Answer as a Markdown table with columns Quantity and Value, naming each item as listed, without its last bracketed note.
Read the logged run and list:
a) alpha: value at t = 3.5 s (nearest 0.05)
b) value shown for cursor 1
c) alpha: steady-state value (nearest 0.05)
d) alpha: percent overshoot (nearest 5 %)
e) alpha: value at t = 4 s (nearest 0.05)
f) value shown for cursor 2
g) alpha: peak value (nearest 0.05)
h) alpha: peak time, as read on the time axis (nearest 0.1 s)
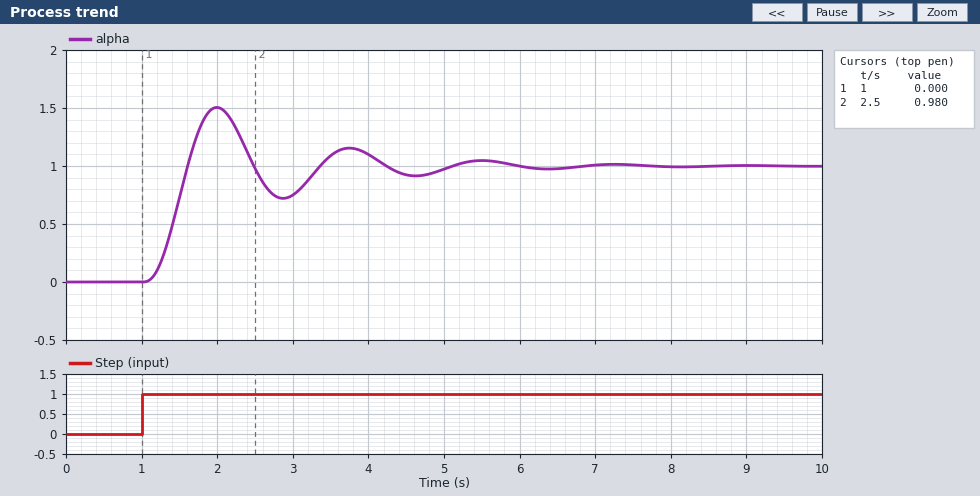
| Quantity | Value |
|---|---|
| alpha: value at t = 3.5 s | 1.10 |
| value shown for cursor 1 | 0.000 |
| alpha: steady-state value | 1.00 |
| alpha: percent overshoot | 50 % |
| alpha: value at t = 4 s | 1.10 |
| value shown for cursor 2 | 0.980 |
| alpha: peak value | 1.50 |
| alpha: peak time, as read on the time axis | 2.0 s |
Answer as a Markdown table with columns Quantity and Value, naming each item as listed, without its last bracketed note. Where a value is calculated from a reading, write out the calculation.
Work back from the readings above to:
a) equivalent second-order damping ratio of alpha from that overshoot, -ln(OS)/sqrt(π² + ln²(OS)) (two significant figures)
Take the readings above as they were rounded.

| Quantity | Value |
|---|---|
| equivalent second-order damping ratio of alpha from that overshoot, -ln(OS)/sqrt(π² + ln²(OS)) | ln(0.5) = -0.693; 0.693 / sqrt(9.870 + 0.480) = 0.22 |
